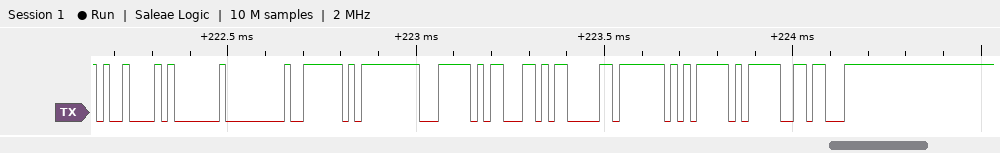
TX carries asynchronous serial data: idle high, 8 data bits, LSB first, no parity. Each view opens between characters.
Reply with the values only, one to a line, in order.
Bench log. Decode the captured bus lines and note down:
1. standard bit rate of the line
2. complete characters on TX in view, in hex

57600 baud
09, 01, 00, 7E, FF, 7C, 63, 83, 7F, 7D, 9F, E3
